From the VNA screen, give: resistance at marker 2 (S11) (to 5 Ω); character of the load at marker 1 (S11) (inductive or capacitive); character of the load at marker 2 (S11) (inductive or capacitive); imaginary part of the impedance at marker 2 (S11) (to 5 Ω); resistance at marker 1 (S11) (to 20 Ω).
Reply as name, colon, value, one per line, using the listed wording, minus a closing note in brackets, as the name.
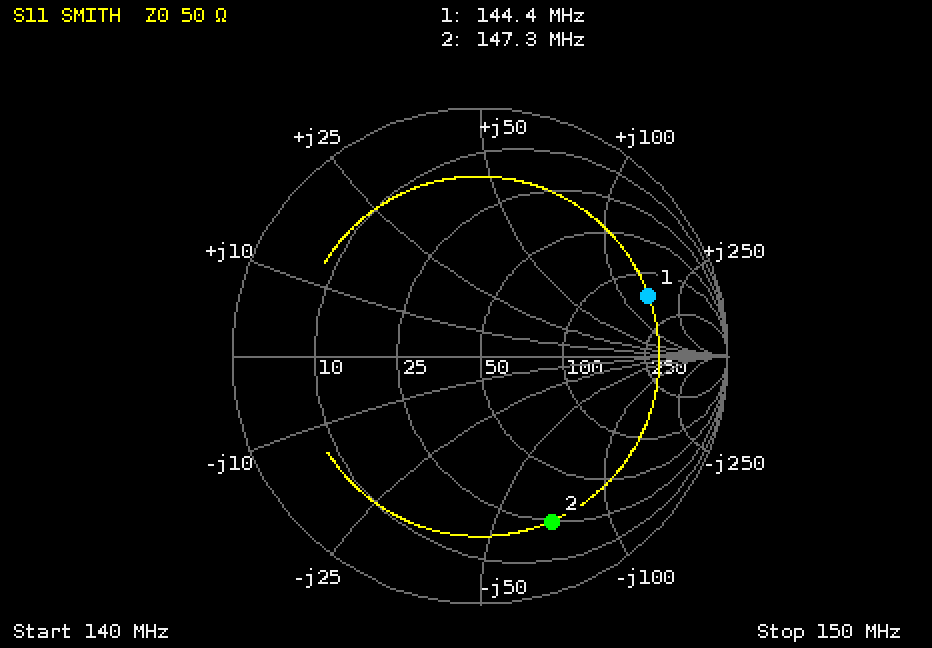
resistance at marker 2 (S11): 25 Ω
character of the load at marker 1 (S11): inductive
character of the load at marker 2 (S11): capacitive
imaginary part of the impedance at marker 2 (S11): -70 Ω
resistance at marker 1 (S11): 140 Ω
